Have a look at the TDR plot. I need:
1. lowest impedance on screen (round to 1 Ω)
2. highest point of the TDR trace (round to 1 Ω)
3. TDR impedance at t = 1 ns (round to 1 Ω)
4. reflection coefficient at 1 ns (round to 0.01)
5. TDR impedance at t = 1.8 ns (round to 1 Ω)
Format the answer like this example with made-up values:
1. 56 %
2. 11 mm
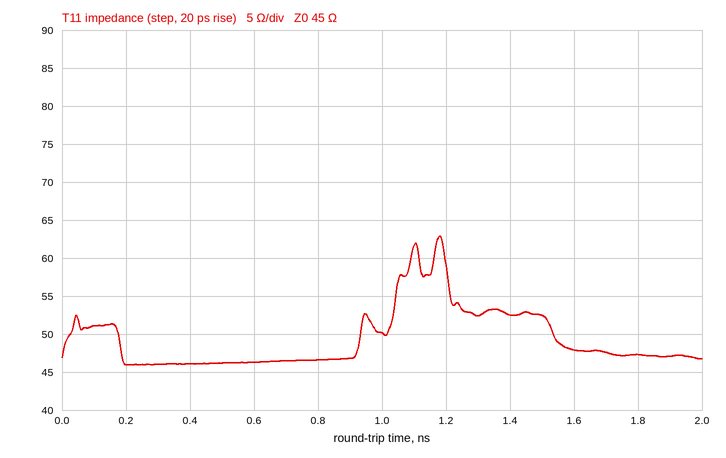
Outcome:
1. 46 Ω
2. 63 Ω
3. 50 Ω
4. +0.05
5. 47 Ω
